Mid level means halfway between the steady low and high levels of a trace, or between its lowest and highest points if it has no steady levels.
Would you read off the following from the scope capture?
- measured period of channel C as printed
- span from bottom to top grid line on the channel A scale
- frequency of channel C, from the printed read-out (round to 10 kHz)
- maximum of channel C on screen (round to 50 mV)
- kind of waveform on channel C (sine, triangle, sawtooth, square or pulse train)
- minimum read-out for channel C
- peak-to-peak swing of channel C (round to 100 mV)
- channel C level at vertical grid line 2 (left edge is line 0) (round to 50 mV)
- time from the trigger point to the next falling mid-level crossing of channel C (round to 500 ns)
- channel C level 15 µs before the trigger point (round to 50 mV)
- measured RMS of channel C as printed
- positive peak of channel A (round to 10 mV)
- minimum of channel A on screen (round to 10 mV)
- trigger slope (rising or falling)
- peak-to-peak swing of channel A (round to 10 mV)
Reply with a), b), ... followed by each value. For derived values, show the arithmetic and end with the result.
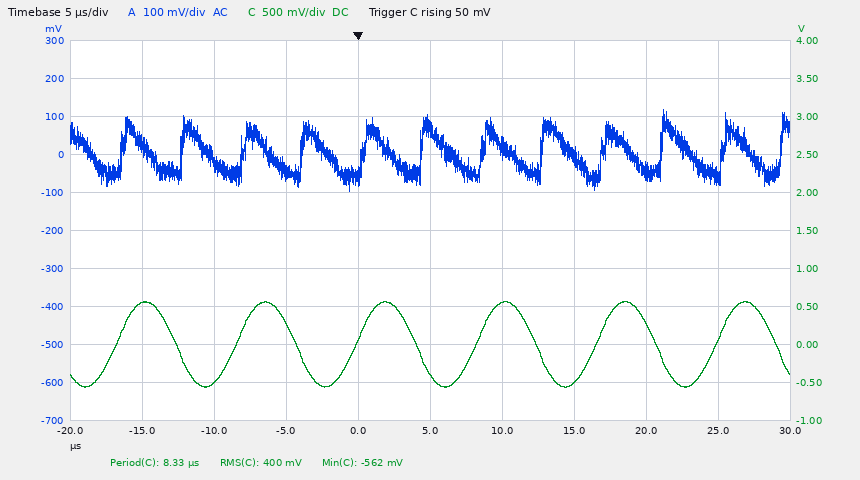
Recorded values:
a) 8.33 µs
b) 1 V
c) 1 / 8.33 µs ≈ 120 kHz
d) 550 mV
e) sine
f) -562 mV
g) 1.10 V
h) -500 mV
i) 4.0 µs
j) 550 mV
k) 400 mV
l) 120 mV
m) -100 mV
n) rising
o) 120 mV − (-100 mV) = 220 mV
